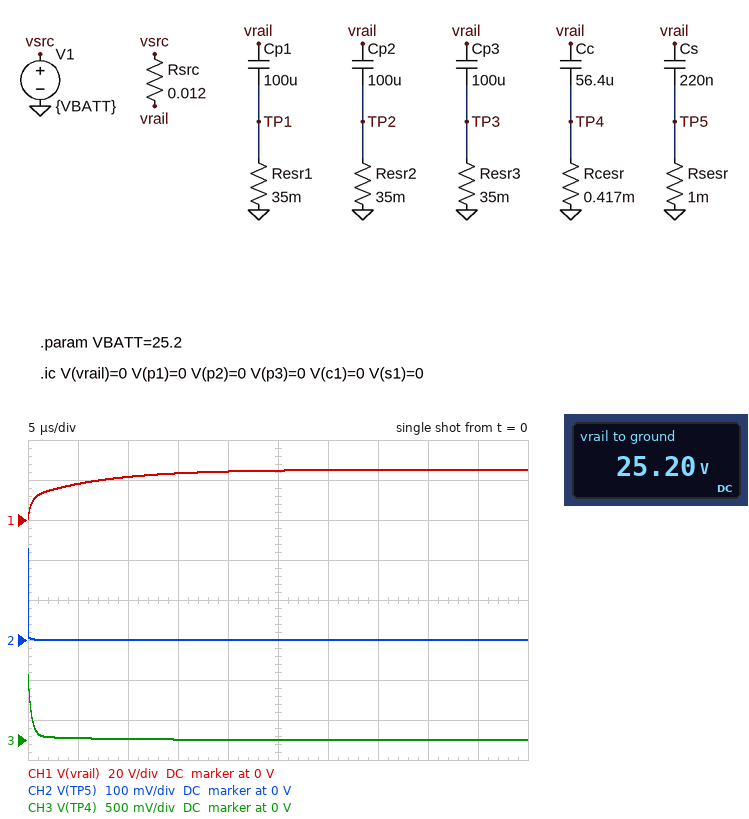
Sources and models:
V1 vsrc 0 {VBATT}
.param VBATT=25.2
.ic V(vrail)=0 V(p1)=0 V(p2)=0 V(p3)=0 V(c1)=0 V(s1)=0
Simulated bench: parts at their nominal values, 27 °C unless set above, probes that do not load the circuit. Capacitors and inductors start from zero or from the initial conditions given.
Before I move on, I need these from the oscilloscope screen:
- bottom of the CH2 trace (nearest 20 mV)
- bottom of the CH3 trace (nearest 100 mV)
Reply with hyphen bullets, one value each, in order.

- 0 V
- 0 V
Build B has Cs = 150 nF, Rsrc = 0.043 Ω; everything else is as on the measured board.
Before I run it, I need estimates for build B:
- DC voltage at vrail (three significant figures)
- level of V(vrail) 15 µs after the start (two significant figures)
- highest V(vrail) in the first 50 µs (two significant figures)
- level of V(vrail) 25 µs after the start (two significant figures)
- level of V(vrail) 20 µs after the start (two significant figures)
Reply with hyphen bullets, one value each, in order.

- 25.2 V
- 16 V
- 24 V
- 20 V
- 18 V
